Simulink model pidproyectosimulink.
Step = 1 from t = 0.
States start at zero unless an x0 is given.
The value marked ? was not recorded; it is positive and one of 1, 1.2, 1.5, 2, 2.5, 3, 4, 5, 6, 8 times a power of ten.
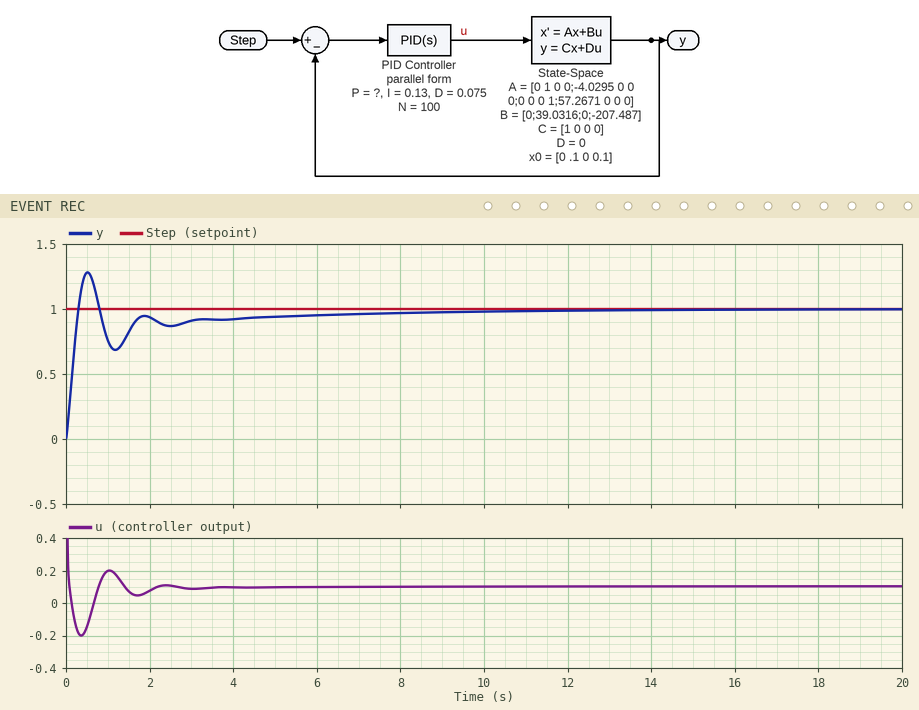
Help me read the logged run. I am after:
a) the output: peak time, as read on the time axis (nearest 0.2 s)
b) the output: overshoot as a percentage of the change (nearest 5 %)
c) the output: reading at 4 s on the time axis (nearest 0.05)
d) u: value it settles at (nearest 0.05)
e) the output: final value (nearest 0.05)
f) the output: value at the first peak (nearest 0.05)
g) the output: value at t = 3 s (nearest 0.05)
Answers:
0.6 s
30 %
0.90
0.10
1.00
1.30
0.90
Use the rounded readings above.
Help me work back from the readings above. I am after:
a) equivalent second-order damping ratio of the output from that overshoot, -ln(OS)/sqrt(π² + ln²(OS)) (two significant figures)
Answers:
0.36
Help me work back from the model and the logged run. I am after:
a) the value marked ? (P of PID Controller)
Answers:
0.5
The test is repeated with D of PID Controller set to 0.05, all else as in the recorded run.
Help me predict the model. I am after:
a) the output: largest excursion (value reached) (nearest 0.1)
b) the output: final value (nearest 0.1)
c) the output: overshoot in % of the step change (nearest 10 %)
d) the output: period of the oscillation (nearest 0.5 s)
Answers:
1.4
1.0
40 %
1.5 s
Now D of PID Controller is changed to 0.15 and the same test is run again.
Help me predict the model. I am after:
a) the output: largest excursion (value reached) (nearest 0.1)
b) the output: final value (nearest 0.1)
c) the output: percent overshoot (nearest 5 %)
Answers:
1.1
1.0
15 %
